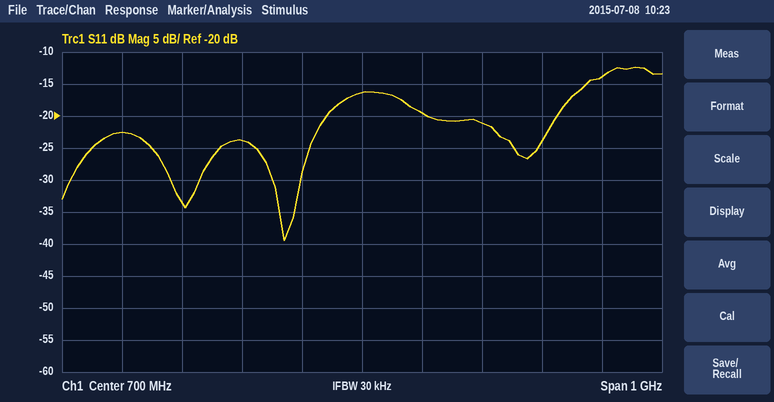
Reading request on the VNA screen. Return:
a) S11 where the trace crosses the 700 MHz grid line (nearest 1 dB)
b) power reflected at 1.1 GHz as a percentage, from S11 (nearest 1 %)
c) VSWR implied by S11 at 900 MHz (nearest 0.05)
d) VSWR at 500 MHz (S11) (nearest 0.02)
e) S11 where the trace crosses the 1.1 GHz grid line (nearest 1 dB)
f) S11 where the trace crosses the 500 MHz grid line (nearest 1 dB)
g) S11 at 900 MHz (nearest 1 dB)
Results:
-16 dB
4 %
1.20
1.14
-14 dB
-24 dB
-21 dB
